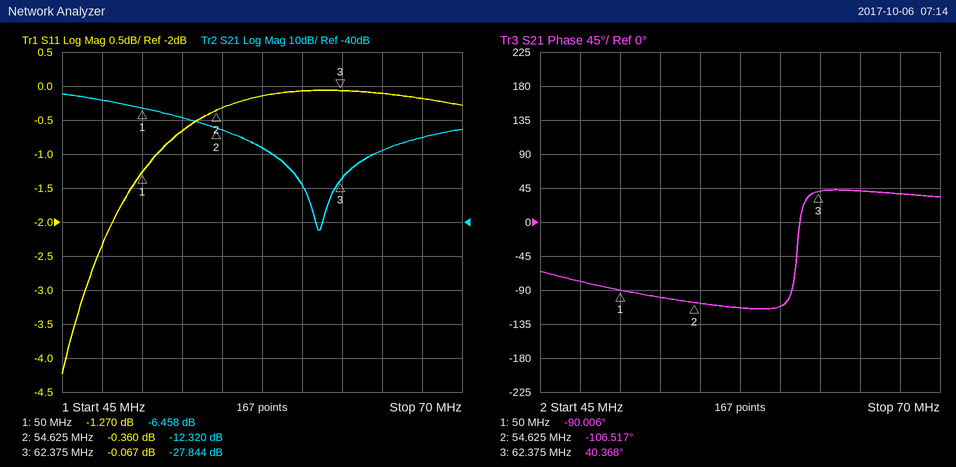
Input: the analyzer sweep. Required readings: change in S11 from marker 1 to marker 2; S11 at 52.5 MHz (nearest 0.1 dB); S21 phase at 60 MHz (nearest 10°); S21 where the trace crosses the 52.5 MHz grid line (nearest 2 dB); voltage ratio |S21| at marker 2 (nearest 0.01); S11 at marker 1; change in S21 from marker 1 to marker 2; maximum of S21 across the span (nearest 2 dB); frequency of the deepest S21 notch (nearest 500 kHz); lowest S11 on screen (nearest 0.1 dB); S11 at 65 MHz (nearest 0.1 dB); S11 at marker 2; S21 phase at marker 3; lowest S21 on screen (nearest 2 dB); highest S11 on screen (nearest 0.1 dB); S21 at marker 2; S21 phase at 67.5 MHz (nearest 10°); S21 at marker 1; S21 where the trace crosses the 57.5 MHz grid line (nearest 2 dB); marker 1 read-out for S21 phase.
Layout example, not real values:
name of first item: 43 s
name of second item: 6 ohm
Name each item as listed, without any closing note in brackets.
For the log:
change in S11 from marker 1 to marker 2: 0.910 dB
S11 at 52.5 MHz: -0.7 dB
S21 phase at 60 MHz: -110°
S21 where the trace crosses the 52.5 MHz grid line: -10 dB
voltage ratio |S21| at marker 2: 0.24
S11 at marker 1: -1.270 dB
change in S21 from marker 1 to marker 2: -5.862 dB
maximum of S21 across the span: -2 dB
frequency of the deepest S21 notch: 61.0 MHz
lowest S11 on screen: -4.2 dB
S11 at 65 MHz: -0.1 dB
S11 at marker 2: -0.360 dB
S21 phase at marker 3: 40.368°
lowest S21 on screen: -42 dB
highest S11 on screen: -0.1 dB
S21 at marker 2: -12.320 dB
S21 phase at 67.5 MHz: 40°
S21 at marker 1: -6.458 dB
S21 where the trace crosses the 57.5 MHz grid line: -18 dB
marker 1 read-out for S21 phase: -90.006°
